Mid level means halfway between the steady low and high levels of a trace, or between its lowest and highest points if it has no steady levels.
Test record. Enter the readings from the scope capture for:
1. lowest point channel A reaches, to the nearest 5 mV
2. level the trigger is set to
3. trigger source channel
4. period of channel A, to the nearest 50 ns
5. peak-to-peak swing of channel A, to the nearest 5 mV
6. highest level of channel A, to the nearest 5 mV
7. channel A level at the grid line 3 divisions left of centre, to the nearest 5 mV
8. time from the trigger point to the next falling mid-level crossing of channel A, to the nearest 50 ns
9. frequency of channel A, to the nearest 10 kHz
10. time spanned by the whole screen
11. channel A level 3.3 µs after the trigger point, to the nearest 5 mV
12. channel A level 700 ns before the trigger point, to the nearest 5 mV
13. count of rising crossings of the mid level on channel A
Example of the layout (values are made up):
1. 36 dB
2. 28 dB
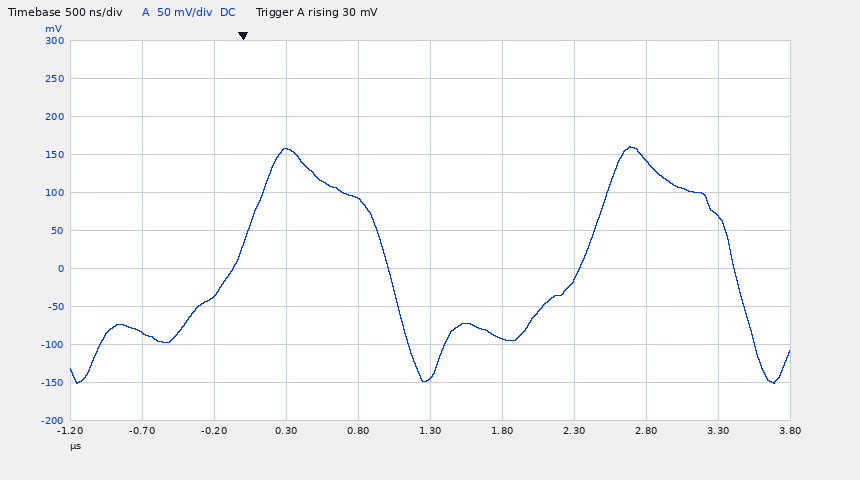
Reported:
1. -150 mV
2. 30 mV
3. channel A
4. 2.40 µs
5. 310 mV
6. 160 mV
7. -35 mV
8. 1.00 µs
9. 420 kHz
10. 5 µs
11. 70 mV
12. -85 mV
13. 2
